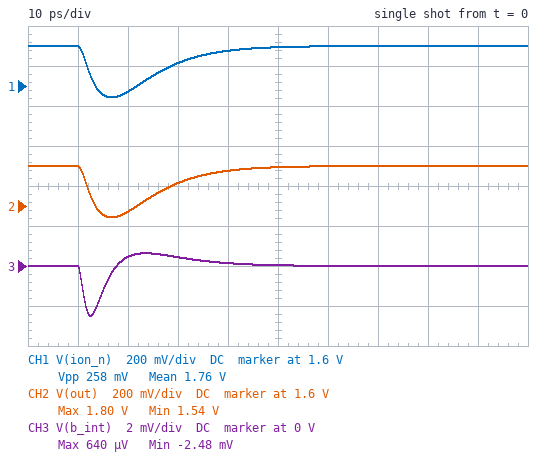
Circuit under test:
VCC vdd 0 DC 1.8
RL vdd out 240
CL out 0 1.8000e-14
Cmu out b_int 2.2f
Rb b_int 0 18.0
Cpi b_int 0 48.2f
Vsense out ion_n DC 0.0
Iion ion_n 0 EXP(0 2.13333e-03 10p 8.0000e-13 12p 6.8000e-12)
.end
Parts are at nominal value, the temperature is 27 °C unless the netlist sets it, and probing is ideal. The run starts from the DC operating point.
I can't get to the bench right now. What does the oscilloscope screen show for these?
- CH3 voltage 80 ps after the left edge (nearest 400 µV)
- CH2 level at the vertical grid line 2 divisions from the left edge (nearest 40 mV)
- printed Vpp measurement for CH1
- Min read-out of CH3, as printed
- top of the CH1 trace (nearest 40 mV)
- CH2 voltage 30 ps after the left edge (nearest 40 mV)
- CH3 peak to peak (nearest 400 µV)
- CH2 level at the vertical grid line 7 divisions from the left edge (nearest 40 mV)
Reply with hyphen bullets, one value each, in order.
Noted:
- 0 V
- 1.56 V
- 258 mV
- -2.48 mV
- 1.80 V
- 1.72 V
- 3.2 mV
- 1.80 V
